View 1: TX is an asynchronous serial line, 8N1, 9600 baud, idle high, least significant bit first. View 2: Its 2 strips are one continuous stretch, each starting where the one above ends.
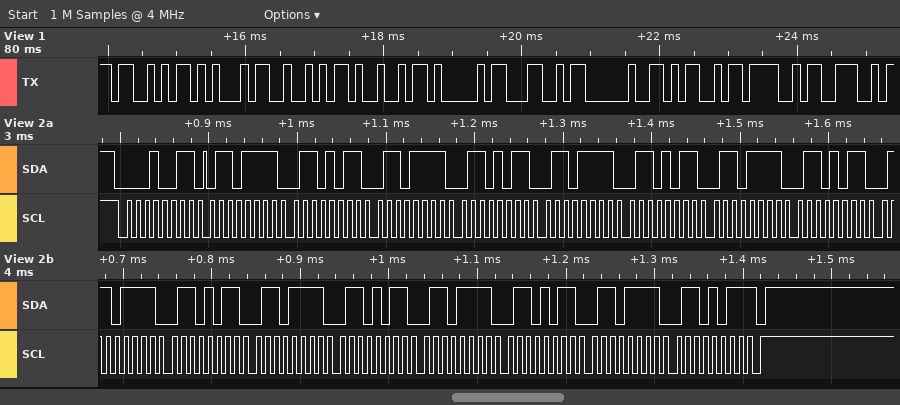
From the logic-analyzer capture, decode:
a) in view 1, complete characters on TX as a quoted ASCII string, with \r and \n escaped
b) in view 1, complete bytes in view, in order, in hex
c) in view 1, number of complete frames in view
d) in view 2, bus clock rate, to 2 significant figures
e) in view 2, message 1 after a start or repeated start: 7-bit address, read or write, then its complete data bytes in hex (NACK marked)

"SERIAL MON"
0x53 0x45 0x52 0x49 0x41 0x4C 0x20 0x4D 0x4F 0x4E
10
100 kHz
0x09 read: 6F 6B 6F 6B 6F 6B 6F 6B 6F 6B 6F 6B 6F 6B 6F 6B NACK
